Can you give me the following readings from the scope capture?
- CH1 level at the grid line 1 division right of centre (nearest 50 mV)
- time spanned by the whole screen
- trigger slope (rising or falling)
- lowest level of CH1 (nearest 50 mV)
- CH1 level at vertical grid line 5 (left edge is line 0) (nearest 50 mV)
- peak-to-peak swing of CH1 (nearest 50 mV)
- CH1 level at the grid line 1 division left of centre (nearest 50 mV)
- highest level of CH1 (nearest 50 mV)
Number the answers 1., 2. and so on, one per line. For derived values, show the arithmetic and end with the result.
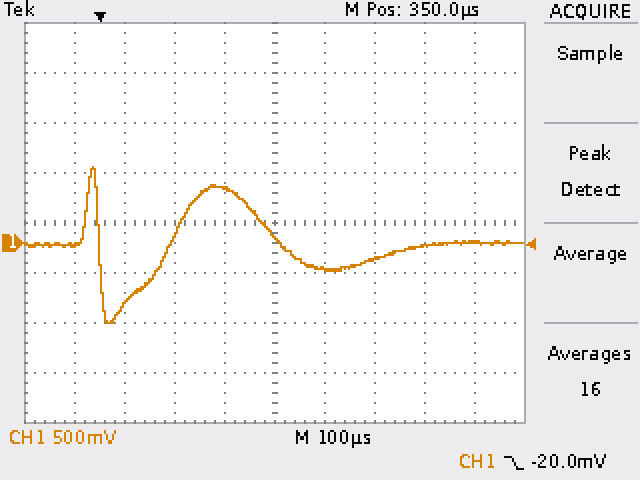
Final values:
1. -250 mV
2. 1 ms
3. falling
4. -800 mV
5. 50 mV
6. 750 mV − (-800 mV) = 1.55 V
7. 550 mV
8. 750 mV
